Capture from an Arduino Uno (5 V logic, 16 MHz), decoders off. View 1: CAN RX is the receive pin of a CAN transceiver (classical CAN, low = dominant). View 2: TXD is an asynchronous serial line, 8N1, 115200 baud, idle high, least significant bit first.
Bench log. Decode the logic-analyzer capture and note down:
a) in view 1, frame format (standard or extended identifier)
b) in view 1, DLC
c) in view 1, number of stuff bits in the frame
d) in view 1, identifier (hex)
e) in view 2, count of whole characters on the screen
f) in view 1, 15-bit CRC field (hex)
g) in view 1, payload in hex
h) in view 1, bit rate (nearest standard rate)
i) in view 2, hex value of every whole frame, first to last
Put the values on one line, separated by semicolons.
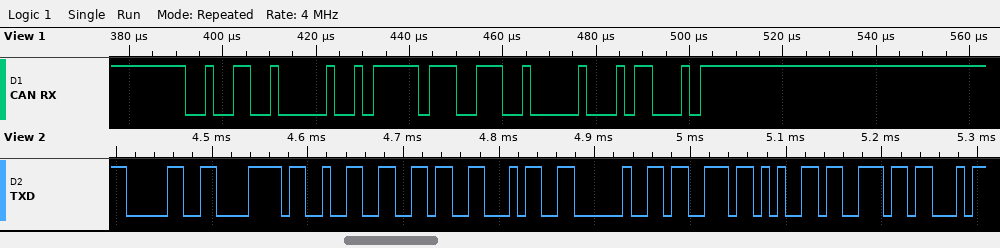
standard; 2; 3; 0x264; 9; 0x0058; FF 39; 500 kbit/s; 30 78 32 36 34 20 73 65 6E
